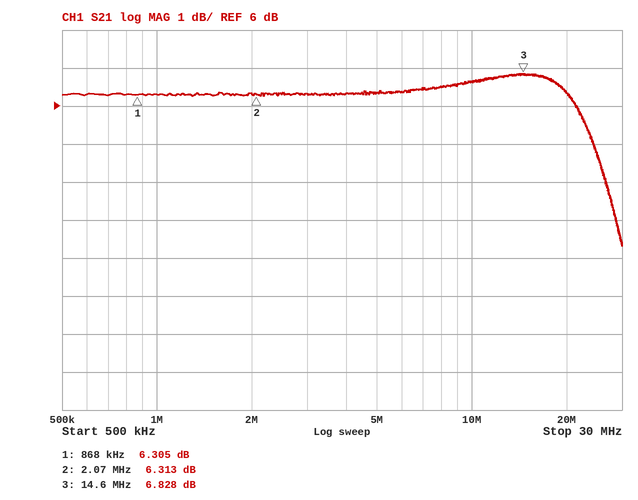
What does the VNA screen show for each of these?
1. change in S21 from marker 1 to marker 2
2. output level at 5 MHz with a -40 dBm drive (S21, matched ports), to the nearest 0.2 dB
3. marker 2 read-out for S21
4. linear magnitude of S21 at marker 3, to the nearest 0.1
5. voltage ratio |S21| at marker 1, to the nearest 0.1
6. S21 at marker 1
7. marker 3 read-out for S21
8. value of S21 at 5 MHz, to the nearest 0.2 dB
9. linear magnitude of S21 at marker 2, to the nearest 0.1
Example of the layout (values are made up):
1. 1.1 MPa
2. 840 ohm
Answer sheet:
1. 0.008 dB
2. -33.6 dBm
3. 6.313 dB
4. 2.2
5. 2.1
6. 6.305 dB
7. 6.828 dB
8. 6.4 dB
9. 2.1
